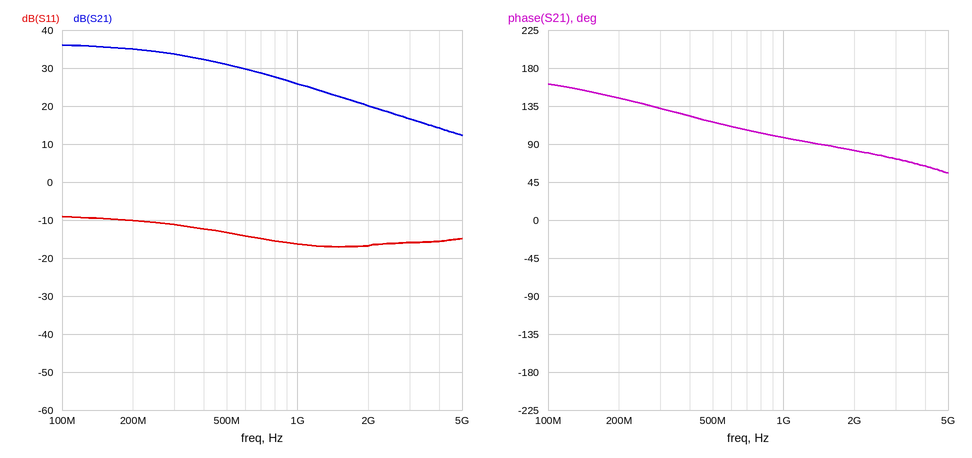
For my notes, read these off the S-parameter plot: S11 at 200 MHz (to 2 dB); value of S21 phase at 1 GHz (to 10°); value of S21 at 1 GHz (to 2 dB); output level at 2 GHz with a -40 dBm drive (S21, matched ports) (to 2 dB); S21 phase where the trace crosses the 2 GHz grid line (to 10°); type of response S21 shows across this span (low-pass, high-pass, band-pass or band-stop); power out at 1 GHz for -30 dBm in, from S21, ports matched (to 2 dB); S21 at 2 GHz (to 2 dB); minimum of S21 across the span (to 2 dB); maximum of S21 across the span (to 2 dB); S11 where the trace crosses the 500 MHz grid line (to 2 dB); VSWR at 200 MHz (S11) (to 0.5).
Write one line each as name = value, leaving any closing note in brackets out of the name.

S11 at 200 MHz = -10 dB
value of S21 phase at 1 GHz = 100°
value of S21 at 1 GHz = 26 dB
output level at 2 GHz with a -40 dBm drive (S21, matched ports) = -20 dBm
S21 phase where the trace crosses the 2 GHz grid line = 80°
type of response S21 shows across this span = low-pass
power out at 1 GHz for -30 dBm in, from S21, ports matched = -4 dBm
S21 at 2 GHz = 20 dB
minimum of S21 across the span = 12 dB
maximum of S21 across the span = 36 dB
S11 where the trace crosses the 500 MHz grid line = -14 dB
VSWR at 200 MHz (S11) = 2.0
